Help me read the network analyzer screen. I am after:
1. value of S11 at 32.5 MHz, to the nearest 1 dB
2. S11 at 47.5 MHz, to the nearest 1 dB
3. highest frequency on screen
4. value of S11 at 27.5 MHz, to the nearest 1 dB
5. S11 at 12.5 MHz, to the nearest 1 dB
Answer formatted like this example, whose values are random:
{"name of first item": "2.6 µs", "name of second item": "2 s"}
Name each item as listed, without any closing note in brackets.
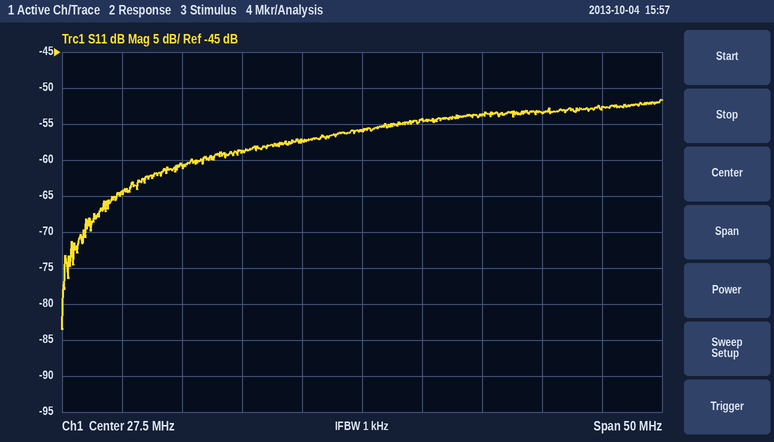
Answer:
{"value of S11 at 32.5 MHz, to the nearest 1 dB": "-54 dB", "S11 at 47.5 MHz, to the nearest 1 dB": "-53 dB", "highest frequency on screen": "52.5 MHz", "value of S11 at 27.5 MHz, to the nearest 1 dB": "-56 dB", "S11 at 12.5 MHz, to the nearest 1 dB": "-61 dB"}
